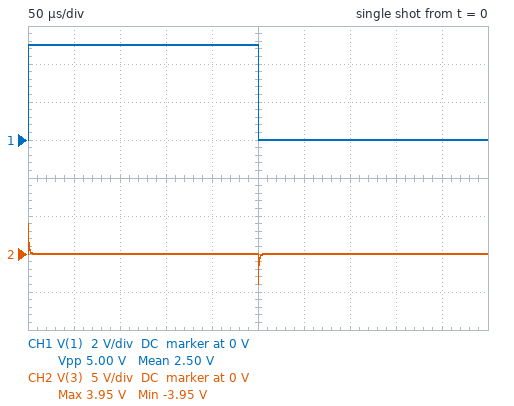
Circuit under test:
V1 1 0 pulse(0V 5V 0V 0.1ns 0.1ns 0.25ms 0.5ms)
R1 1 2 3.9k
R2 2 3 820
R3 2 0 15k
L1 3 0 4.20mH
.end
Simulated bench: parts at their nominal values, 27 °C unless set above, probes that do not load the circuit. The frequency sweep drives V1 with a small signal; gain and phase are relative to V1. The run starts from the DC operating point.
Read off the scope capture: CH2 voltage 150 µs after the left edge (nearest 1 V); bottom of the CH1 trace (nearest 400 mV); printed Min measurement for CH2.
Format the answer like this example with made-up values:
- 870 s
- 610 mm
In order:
- 0 V
- 0 V
- -3.95 V
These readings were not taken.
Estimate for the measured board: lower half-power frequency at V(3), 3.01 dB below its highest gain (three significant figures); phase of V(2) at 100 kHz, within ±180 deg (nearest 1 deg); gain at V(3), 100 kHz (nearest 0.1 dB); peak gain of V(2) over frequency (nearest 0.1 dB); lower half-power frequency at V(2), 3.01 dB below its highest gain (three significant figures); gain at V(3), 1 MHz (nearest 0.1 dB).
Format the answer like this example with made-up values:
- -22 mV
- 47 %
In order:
- 148 kHz
- 39 deg
- -7.1 dB
- -2.0 dB
- 142 kHz
- -2.1 dB
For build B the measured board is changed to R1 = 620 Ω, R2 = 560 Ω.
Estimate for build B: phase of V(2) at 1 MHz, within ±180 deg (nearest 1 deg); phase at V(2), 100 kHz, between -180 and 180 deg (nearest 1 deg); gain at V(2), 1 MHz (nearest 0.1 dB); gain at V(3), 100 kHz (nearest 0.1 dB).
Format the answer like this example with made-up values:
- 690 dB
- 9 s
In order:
- 1 deg
- 12 deg
- -0.4 dB
- -1.1 dB
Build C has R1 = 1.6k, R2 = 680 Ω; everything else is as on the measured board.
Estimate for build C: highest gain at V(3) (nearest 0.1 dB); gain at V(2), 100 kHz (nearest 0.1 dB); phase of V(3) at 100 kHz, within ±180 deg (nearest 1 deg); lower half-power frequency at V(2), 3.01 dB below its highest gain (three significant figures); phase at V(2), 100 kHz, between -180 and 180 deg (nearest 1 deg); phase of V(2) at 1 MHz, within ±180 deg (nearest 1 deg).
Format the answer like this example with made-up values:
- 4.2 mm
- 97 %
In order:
- -0.9 dB
- -2.8 dB
- 39 deg
- 71.8 kHz
- 24 deg
- 3 deg
